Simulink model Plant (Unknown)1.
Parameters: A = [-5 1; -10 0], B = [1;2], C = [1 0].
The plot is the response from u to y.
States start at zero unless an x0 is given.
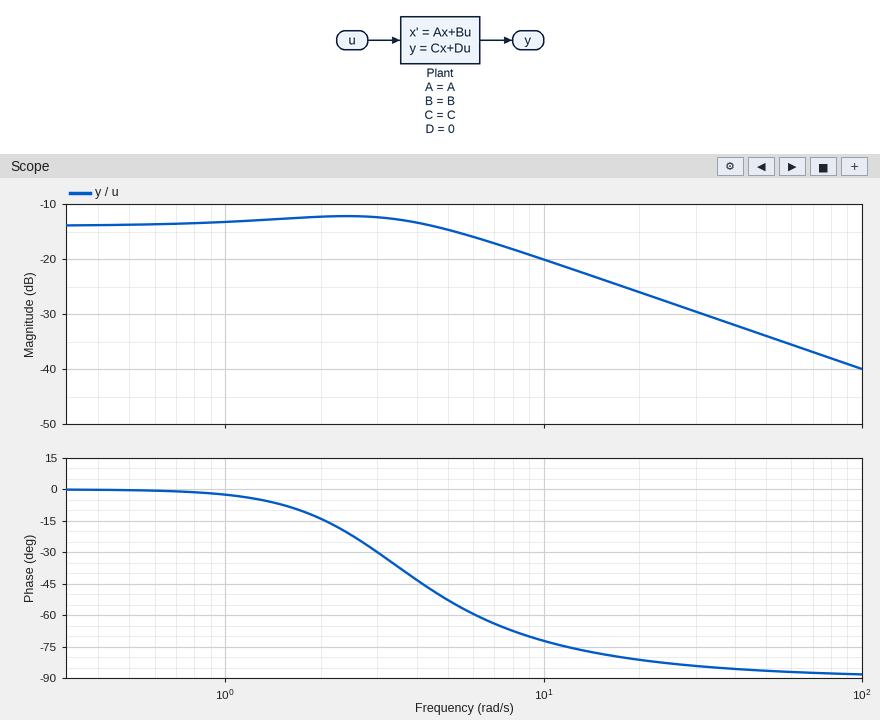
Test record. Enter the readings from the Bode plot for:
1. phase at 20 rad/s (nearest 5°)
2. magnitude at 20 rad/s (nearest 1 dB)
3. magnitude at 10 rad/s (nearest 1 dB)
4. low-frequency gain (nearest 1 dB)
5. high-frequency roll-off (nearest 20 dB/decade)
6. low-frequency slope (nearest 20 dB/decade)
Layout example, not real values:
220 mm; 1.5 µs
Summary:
-80°; -26 dB; -20 dB; -14 dB; -20 dB/decade; 0 dB/decade
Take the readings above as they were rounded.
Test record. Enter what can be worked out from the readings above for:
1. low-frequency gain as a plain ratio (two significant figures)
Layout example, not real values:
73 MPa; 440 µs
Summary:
0.20
